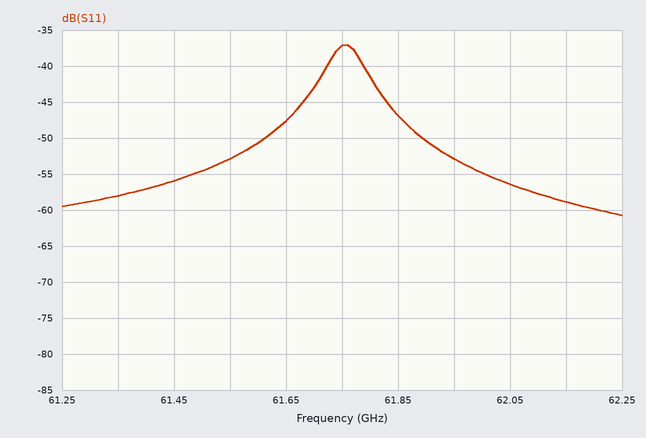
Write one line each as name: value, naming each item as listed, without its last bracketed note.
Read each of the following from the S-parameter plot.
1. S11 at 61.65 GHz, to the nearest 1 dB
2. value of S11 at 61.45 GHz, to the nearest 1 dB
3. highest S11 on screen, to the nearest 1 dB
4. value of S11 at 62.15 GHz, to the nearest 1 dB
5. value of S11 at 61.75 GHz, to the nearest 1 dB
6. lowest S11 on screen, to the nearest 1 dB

S11 at 61.65 GHz, to the nearest 1 dB: -48 dB
value of S11 at 61.45 GHz, to the nearest 1 dB: -56 dB
highest S11 on screen, to the nearest 1 dB: -37 dB
value of S11 at 62.15 GHz, to the nearest 1 dB: -59 dB
value of S11 at 61.75 GHz, to the nearest 1 dB: -37 dB
lowest S11 on screen, to the nearest 1 dB: -61 dB
